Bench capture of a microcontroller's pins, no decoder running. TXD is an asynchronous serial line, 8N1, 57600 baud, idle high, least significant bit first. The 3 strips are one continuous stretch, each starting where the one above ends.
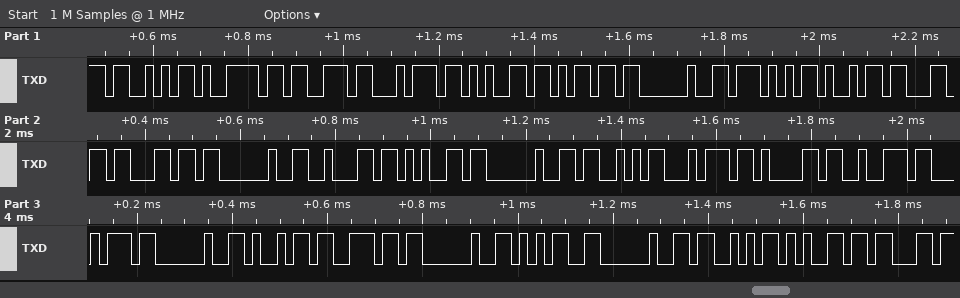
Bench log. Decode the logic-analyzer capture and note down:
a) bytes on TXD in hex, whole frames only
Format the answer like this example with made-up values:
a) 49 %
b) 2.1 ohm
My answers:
a) 53 79 73 74 65 6D 20 57 69 6C 6C 20 62 65 20 53 74 61 72 74 20 69 6E 20 35 20 53 65 63
